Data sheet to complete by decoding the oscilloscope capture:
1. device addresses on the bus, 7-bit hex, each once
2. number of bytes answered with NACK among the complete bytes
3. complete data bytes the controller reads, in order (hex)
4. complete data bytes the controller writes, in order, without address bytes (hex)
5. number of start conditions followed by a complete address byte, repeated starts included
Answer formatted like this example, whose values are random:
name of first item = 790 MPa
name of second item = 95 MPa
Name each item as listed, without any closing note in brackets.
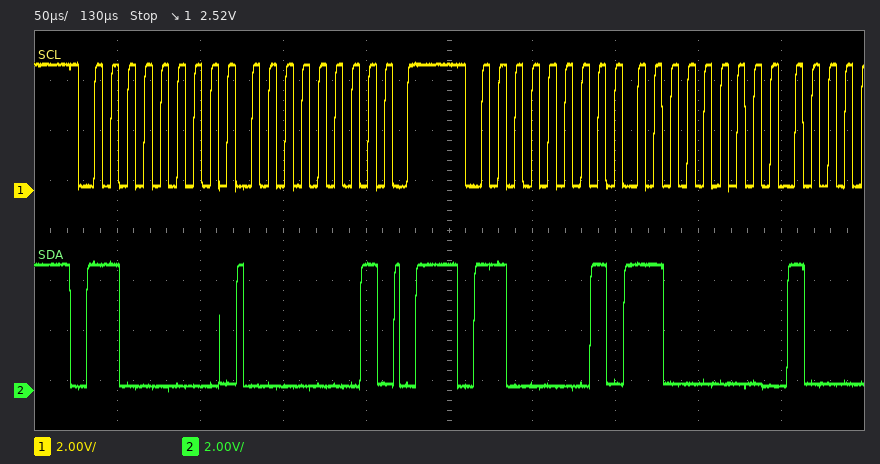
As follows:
device addresses on the bus, 7-bit hex, each once = 0x60
number of bytes answered with NACK among the complete bytes = 0
complete data bytes the controller reads, in order = C0
complete data bytes the controller writes, in order, without address bytes = 01
number of start conditions followed by a complete address byte, repeated starts included = 2
